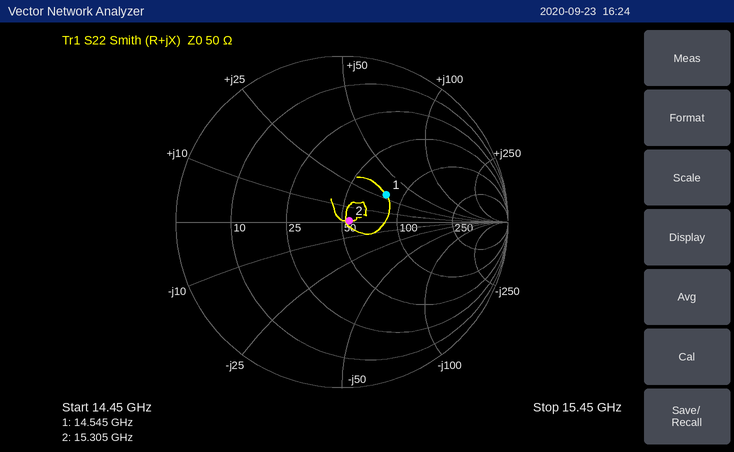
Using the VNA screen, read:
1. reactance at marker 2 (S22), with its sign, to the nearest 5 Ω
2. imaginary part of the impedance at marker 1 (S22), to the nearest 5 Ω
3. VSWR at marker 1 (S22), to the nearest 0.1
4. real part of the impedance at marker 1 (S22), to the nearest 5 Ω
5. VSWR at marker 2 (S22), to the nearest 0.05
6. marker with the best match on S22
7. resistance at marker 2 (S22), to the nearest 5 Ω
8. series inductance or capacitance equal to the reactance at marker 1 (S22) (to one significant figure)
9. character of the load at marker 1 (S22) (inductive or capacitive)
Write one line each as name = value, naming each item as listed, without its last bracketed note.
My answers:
reactance at marker 2 (S22), with its sign, to the nearest 5 Ω = 0 Ω
imaginary part of the impedance at marker 1 (S22), to the nearest 5 Ω = +30 Ω
VSWR at marker 1 (S22), to the nearest 0.1 = 1.9
real part of the impedance at marker 1 (S22), to the nearest 5 Ω = 80 Ω
VSWR at marker 2 (S22), to the nearest 0.05 = 1.10
marker with the best match on S22 = marker 2
resistance at marker 2 (S22), to the nearest 5 Ω = 55 Ω
series inductance or capacitance equal to the reactance at marker 1 (S22) = 300 pH
character of the load at marker 1 (S22) = inductive
